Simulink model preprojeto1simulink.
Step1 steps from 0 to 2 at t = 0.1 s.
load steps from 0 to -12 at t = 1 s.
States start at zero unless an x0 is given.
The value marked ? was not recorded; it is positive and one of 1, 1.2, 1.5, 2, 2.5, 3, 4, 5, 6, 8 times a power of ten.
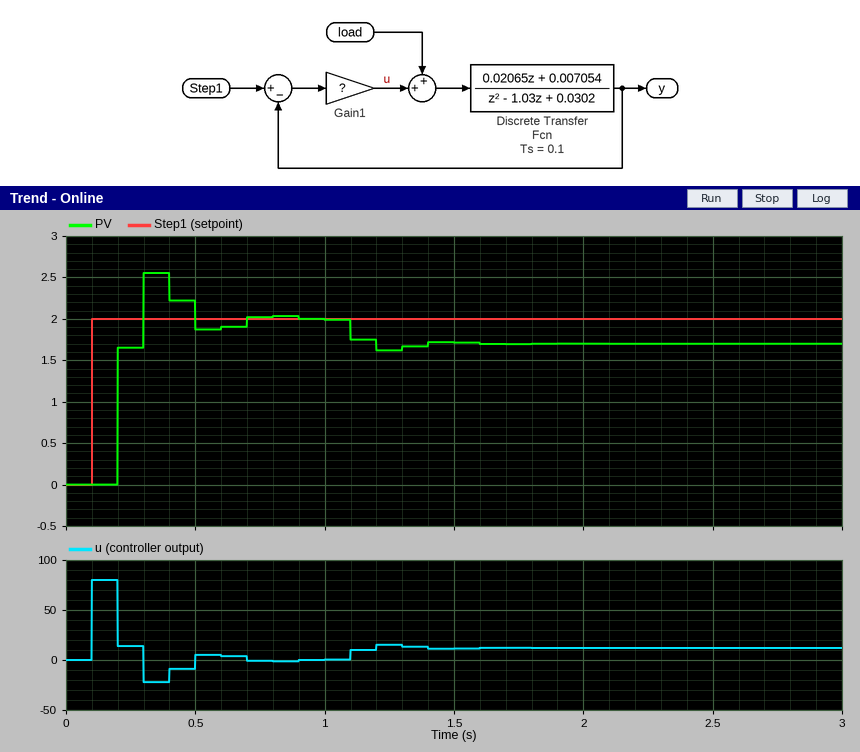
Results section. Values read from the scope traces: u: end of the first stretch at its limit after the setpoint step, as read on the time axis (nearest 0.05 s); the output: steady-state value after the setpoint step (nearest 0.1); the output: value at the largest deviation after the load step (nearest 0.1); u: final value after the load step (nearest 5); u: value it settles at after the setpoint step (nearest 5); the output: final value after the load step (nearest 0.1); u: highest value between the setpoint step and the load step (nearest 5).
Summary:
0.20 s
2.0
1.6
10
0
1.7
80
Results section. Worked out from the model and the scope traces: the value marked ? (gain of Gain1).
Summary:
40
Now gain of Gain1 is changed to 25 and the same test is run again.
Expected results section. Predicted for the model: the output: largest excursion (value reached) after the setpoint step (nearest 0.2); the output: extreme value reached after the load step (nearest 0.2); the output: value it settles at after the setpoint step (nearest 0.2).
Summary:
2.2
1.4
2.0
